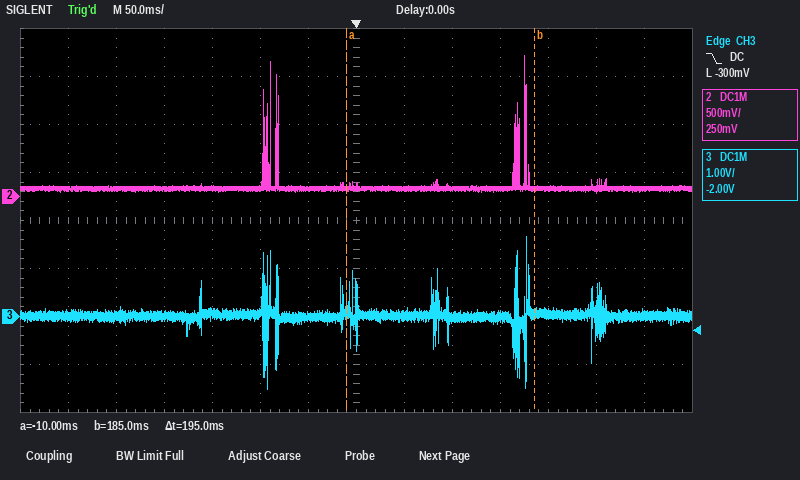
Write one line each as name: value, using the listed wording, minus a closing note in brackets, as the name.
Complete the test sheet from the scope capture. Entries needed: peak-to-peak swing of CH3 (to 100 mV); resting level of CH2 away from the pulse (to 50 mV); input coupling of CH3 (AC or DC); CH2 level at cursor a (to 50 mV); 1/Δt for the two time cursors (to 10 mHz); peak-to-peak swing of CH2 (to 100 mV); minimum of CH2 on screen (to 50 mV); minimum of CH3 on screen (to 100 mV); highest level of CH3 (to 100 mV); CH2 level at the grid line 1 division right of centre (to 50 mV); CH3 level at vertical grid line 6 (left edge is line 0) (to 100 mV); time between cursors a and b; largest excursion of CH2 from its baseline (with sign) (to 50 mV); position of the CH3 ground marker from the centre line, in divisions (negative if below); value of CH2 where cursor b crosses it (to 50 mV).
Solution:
peak-to-peak swing of CH3: 3.2 V
resting level of CH2 away from the pulse: 100 mV
input coupling of CH3: DC
CH2 level at cursor a: 100 mV
1/Δt for the two time cursors: 5.13 Hz
peak-to-peak swing of CH2: 1.40 V
minimum of CH2 on screen: 50 mV
minimum of CH3 on screen: -1.5 V
highest level of CH3: 1.7 V
CH2 level at the grid line 1 division right of centre: 100 mV
CH3 level at vertical grid line 6 (left edge is line 0): 0.0 V
time between cursors a and b: 195 ms
largest excursion of CH2 from its baseline (with sign): +1.40 V
position of the CH3 ground marker from the centre line, in divisions: -2.0 div
value of CH2 where cursor b crosses it: 100 mV
